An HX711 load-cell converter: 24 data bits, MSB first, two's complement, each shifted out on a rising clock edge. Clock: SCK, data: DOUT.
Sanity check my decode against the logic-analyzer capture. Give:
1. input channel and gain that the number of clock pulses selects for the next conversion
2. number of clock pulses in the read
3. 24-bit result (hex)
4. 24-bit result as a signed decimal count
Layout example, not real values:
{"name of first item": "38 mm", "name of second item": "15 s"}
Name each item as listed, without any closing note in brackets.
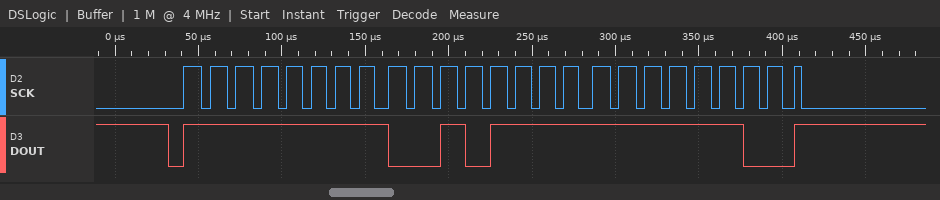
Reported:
{"input channel and gain that the number of clock pulses selects for the next conversion": "channel A, gain 128", "number of clock pulses in the read": "25", "24-bit result": "0xFF2FFC", "24-bit result as a signed decimal count": "-53252"}
